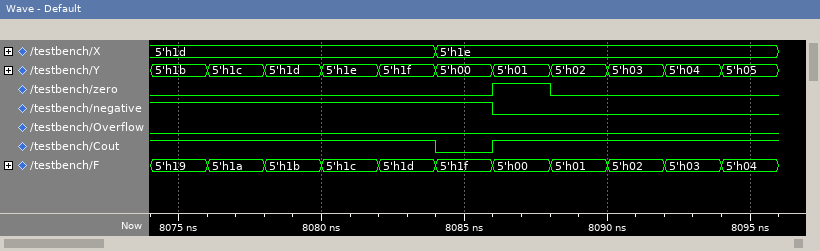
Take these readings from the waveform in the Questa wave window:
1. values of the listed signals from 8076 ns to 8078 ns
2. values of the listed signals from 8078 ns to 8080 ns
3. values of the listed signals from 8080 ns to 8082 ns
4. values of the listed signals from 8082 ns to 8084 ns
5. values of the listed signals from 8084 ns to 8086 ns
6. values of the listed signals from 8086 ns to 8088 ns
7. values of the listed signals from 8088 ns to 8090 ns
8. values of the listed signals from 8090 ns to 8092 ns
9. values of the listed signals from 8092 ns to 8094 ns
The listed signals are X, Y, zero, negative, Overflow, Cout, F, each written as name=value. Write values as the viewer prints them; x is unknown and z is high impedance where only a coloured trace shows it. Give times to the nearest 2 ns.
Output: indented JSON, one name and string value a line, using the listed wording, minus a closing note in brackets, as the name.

{
  "values of the listed signals from 8076 ns to 8078 ns": "X=5'h1d, Y=5'h1c, zero=0, negative=1, Overflow=0, Cout=1, F=5'h1a",
  "values of the listed signals from 8078 ns to 8080 ns": "X=5'h1d, Y=5'h1d, zero=0, negative=1, Overflow=0, Cout=1, F=5'h1b",
  "values of the listed signals from 8080 ns to 8082 ns": "X=5'h1d, Y=5'h1e, zero=0, negative=1, Overflow=0, Cout=1, F=5'h1c",
  "values of the listed signals from 8082 ns to 8084 ns": "X=5'h1d, Y=5'h1f, zero=0, negative=1, Overflow=0, Cout=1, F=5'h1d",
  "values of the listed signals from 8084 ns to 8086 ns": "X=5'h1e, Y=5'h00, zero=0, negative=1, Overflow=0, Cout=0, F=5'h1f",
  "values of the listed signals from 8086 ns to 8088 ns": "X=5'h1e, Y=5'h01, zero=1, negative=0, Overflow=0, Cout=1, F=5'h00",
  "values of the listed signals from 8088 ns to 8090 ns": "X=5'h1e, Y=5'h02, zero=0, negative=0, Overflow=0, Cout=1, F=5'h01",
  "values of the listed signals from 8090 ns to 8092 ns": "X=5'h1e, Y=5'h03, zero=0, negative=0, Overflow=0, Cout=1, F=5'h02",
  "values of the listed signals from 8092 ns to 8094 ns": "X=5'h1e, Y=5'h04, zero=0, negative=0, Overflow=0, Cout=1, F=5'h03"
}
